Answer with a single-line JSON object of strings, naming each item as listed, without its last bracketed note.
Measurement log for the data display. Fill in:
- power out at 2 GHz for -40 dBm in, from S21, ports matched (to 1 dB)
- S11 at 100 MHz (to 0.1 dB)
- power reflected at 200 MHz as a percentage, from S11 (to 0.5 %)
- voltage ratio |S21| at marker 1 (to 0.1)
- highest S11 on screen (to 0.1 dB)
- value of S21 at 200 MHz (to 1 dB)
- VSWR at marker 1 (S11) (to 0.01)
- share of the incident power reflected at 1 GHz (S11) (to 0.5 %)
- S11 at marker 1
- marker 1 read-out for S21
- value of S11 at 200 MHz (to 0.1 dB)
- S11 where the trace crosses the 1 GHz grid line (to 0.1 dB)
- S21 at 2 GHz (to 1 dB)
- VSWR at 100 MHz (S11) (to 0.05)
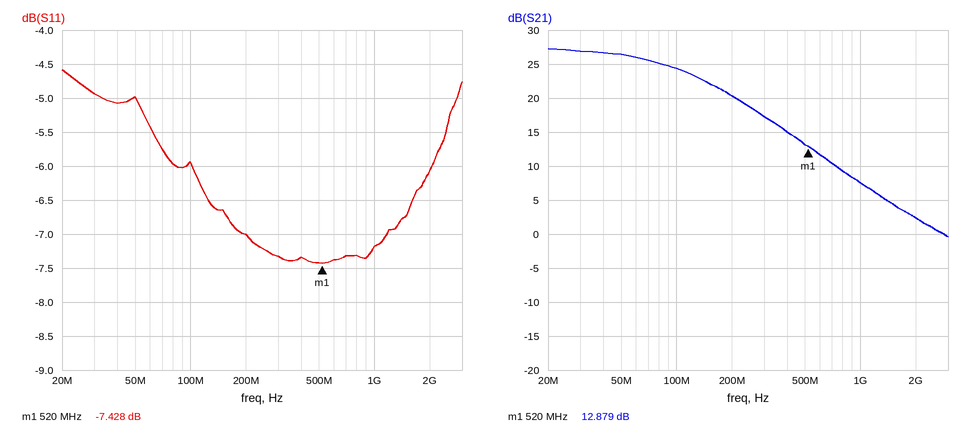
{"power out at 2 GHz for -40 dBm in, from S21, ports matched": "-38 dBm", "S11 at 100 MHz": "-5.9 dB", "power reflected at 200 MHz as a percentage, from S11": "20.0 %", "voltage ratio |S21| at marker 1": "4.4", "highest S11 on screen": "-4.6 dB", "value of S21 at 200 MHz": "20 dB", "VSWR at marker 1 (S11)": "2.48", "share of the incident power reflected at 1 GHz (S11)": "19.0 %", "S11 at marker 1": "-7.428 dB", "marker 1 read-out for S21": "12.879 dB", "value of S11 at 200 MHz": "-7.0 dB", "S11 where the trace crosses the 1 GHz grid line": "-7.2 dB", "S21 at 2 GHz": "2 dB", "VSWR at 100 MHz (S11)": "3.05"}
